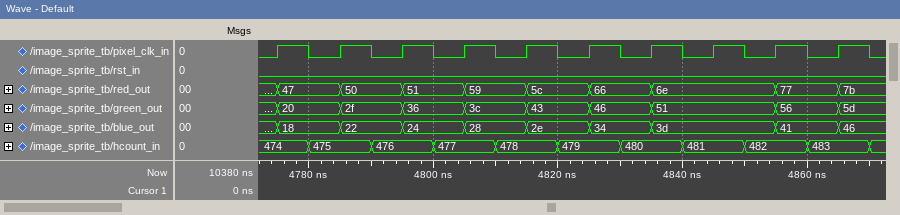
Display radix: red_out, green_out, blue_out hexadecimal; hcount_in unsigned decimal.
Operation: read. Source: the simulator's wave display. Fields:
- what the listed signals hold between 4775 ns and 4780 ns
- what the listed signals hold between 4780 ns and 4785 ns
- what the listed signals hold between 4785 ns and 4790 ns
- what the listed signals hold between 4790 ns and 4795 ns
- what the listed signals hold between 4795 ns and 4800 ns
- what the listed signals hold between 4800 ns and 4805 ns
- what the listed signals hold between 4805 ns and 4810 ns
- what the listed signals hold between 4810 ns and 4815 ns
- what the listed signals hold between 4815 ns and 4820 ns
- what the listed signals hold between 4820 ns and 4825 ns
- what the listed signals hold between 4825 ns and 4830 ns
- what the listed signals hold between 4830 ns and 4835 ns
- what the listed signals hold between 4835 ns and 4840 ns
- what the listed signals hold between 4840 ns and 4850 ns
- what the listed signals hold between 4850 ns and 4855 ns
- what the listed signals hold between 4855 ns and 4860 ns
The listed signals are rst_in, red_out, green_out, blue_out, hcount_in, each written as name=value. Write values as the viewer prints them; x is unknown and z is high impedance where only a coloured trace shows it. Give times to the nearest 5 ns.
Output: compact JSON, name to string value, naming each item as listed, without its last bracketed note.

{"what the listed signals hold between 4775 ns and 4780 ns": "rst_in=0, red_out=47, green_out=20, blue_out=18, hcount_in=474", "what the listed signals hold between 4780 ns and 4785 ns": "rst_in=0, red_out=47, green_out=20, blue_out=18, hcount_in=475", "what the listed signals hold between 4785 ns and 4790 ns": "rst_in=0, red_out=50, green_out=2f, blue_out=22, hcount_in=475", "what the listed signals hold between 4790 ns and 4795 ns": "rst_in=0, red_out=50, green_out=2f, blue_out=22, hcount_in=476", "what the listed signals hold between 4795 ns and 4800 ns": "rst_in=0, red_out=51, green_out=36, blue_out=24, hcount_in=476", "what the listed signals hold between 4800 ns and 4805 ns": "rst_in=0, red_out=51, green_out=36, blue_out=24, hcount_in=477", "what the listed signals hold between 4805 ns and 4810 ns": "rst_in=0, red_out=59, green_out=3c, blue_out=28, hcount_in=477", "what the listed signals hold between 4810 ns and 4815 ns": "rst_in=0, red_out=59, green_out=3c, blue_out=28, hcount_in=478", "what the listed signals hold between 4815 ns and 4820 ns": "rst_in=0, red_out=5c, green_out=43, blue_out=2e, hcount_in=478", "what the listed signals hold between 4820 ns and 4825 ns": "rst_in=0, red_out=5c, green_out=43, blue_out=2e, hcount_in=479", "what the listed signals hold between 4825 ns and 4830 ns": "rst_in=0, red_out=66, green_out=46, blue_out=34, hcount_in=479", "what the listed signals hold between 4830 ns and 4835 ns": "rst_in=0, red_out=66, green_out=46, blue_out=34, hcount_in=480", "what the listed signals hold between 4835 ns and 4840 ns": "rst_in=0, red_out=6e, green_out=51, blue_out=3d, hcount_in=480", "what the listed signals hold between 4840 ns and 4850 ns": "rst_in=0, red_out=6e, green_out=51, blue_out=3d, hcount_in=481", "what the listed signals hold between 4850 ns and 4855 ns": "rst_in=0, red_out=6e, green_out=51, blue_out=3d, hcount_in=482", "what the listed signals hold between 4855 ns and 4860 ns": "rst_in=0, red_out=77, green_out=56, blue_out=41, hcount_in=482"}
